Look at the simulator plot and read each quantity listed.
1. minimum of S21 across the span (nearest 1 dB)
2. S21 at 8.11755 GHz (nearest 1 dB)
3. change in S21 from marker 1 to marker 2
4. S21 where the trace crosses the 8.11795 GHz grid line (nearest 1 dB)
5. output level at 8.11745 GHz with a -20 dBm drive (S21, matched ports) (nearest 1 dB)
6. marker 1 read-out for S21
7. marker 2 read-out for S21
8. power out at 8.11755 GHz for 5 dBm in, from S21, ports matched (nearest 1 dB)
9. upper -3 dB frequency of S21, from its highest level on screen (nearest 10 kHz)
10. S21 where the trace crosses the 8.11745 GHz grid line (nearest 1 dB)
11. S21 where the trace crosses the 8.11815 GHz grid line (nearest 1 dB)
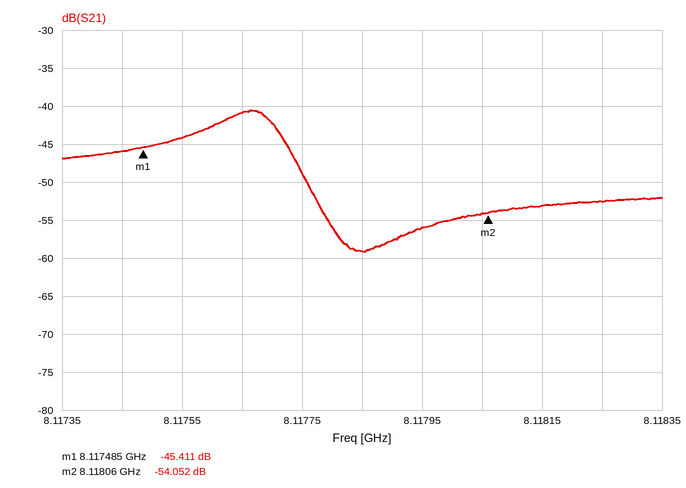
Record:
-59 dB
-44 dB
-8.641 dB
-56 dB
-66 dBm
-45.411 dB
-54.052 dB
-39 dBm
8.11771 GHz
-46 dB
-53 dB
